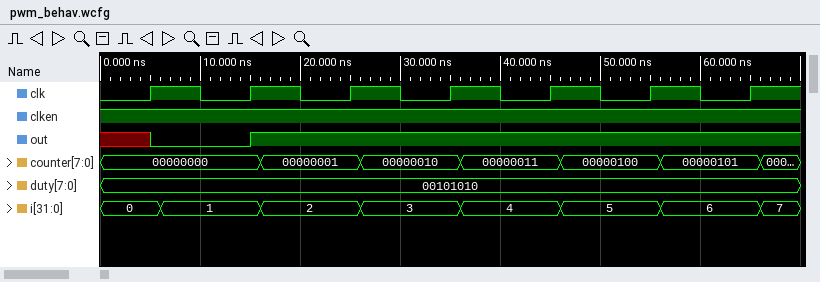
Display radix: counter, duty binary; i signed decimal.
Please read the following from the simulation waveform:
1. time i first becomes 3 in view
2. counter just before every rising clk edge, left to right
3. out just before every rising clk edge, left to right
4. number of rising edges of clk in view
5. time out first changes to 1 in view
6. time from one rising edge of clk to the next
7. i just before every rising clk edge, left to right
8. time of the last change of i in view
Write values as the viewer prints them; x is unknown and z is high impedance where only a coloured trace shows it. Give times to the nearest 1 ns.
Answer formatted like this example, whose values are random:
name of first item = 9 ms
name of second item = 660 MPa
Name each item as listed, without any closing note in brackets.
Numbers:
time i first becomes 3 in view = 26 ns
counter just before every rising clk edge, left to right = 00000000, 00000000, 00000001, 00000010, 00000011, 00000100, 00000101
out just before every rising clk edge, left to right = x 0 1 1 1 1 1
number of rising edges of clk in view = 7
time out first changes to 1 in view = 15 ns
time from one rising edge of clk to the next = 10 ns
i just before every rising clk edge, left to right = 0, 1, 2, 3, 4, 5, 6
time of the last change of i in view = 66 ns
